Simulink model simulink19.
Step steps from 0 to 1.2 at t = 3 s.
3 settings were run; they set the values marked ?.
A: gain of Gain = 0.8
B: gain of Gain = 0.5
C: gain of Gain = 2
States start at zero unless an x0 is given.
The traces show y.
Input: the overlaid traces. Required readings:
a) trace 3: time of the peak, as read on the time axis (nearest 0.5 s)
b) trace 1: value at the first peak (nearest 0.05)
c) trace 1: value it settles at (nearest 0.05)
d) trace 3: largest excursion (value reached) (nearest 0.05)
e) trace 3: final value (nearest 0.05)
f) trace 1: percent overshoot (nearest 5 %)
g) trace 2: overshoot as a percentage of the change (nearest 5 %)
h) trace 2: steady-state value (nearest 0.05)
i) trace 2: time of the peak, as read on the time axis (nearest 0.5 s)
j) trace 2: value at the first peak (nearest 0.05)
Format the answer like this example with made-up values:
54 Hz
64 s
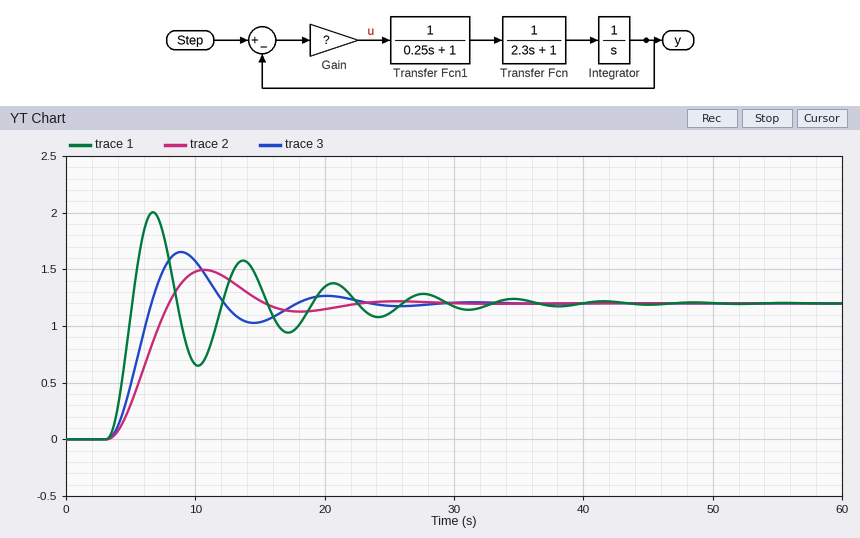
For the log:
9.0 s
2.00
1.20
1.65
1.20
65 %
25 %
1.20
10.5 s
1.50
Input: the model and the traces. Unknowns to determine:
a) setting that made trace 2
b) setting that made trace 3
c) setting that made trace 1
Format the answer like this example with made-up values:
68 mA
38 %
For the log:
B
A
C
